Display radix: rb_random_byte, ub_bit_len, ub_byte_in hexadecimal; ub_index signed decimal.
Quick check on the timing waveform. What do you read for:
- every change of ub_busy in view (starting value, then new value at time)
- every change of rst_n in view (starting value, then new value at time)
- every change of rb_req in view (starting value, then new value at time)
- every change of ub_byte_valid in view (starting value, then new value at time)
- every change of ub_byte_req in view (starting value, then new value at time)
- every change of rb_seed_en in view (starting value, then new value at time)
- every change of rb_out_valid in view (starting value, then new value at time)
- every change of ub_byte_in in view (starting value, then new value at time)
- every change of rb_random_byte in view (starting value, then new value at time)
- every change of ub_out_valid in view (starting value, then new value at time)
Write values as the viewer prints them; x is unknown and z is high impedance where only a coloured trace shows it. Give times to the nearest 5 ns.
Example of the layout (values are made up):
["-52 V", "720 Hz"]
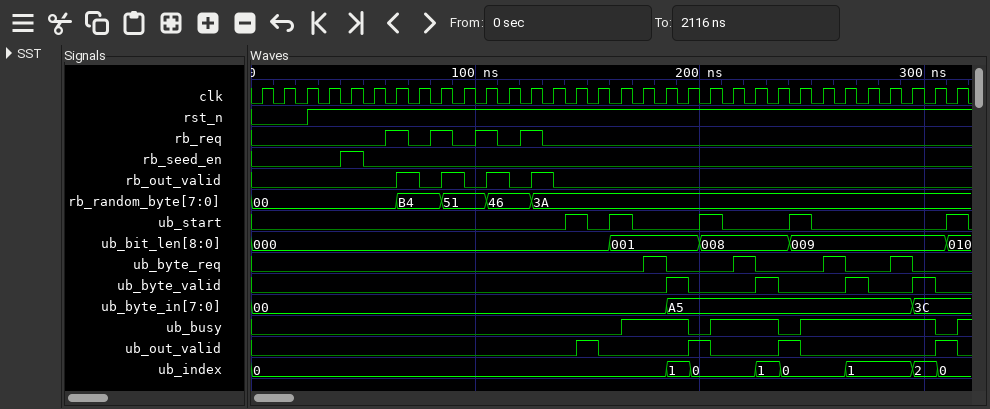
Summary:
["0, 1 at 165 ns, 0 at 195 ns, 1 at 205 ns, 0 at 235 ns, 1 at 245 ns, 0 at 305 ns, 1 at 315 ns", "0, 1 at 25 ns", "0, 1 at 60 ns, 0 at 70 ns, 1 at 80 ns, 0 at 90 ns, 1 at 100 ns, 0 at 110 ns, 1 at 120 ns, 0 at 130 ns", "0, 1 at 185 ns, 0 at 195 ns, 1 at 225 ns, 0 at 235 ns, 1 at 265 ns, 0 at 275 ns, 1 at 295 ns, 0 at 305 ns", "0, 1 at 175 ns, 0 at 185 ns, 1 at 215 ns, 0 at 225 ns, 1 at 255 ns, 0 at 265 ns, 1 at 285 ns, 0 at 295 ns", "0, 1 at 40 ns, 0 at 50 ns", "0, 1 at 65 ns, 0 at 75 ns, 1 at 85 ns, 0 at 95 ns, 1 at 105 ns, 0 at 115 ns, 1 at 125 ns, 0 at 135 ns", "00, A5 at 185 ns, 3C at 295 ns", "00, B4 at 65 ns, 51 at 85 ns, 46 at 105 ns, 3A at 125 ns", "0, 1 at 145 ns, 0 at 155 ns, 1 at 195 ns, 0 at 205 ns, 1 at 235 ns, 0 at 245 ns, 1 at 305 ns, 0 at 315 ns"]
